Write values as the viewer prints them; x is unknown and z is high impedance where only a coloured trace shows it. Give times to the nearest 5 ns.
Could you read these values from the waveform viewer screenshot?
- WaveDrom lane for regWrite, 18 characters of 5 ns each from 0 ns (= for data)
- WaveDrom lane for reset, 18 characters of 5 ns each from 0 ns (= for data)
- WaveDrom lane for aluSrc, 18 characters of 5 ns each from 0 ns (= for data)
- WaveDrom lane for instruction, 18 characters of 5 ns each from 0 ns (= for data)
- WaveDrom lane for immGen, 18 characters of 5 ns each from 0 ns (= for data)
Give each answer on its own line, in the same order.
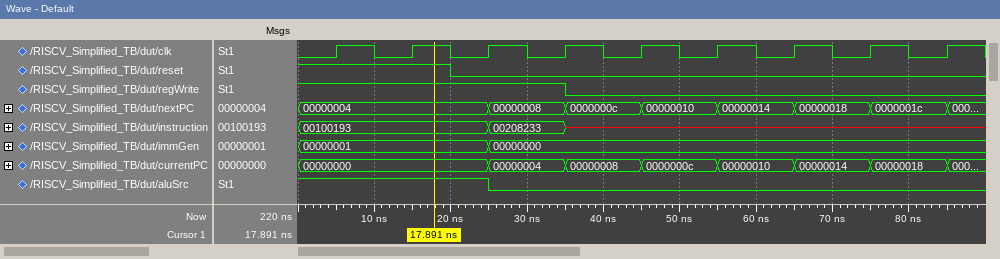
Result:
{name: 'regWrite', wave: '1......0..........'}
{name: 'reset', wave: '1...0.............'}
{name: 'aluSrc', wave: '1....0............'}
{name: 'instruction', wave: '=....=.x..........', data: '00100193 00208233'}
{name: 'immGen', wave: '=....=............', data: '00000001 00000000'}
